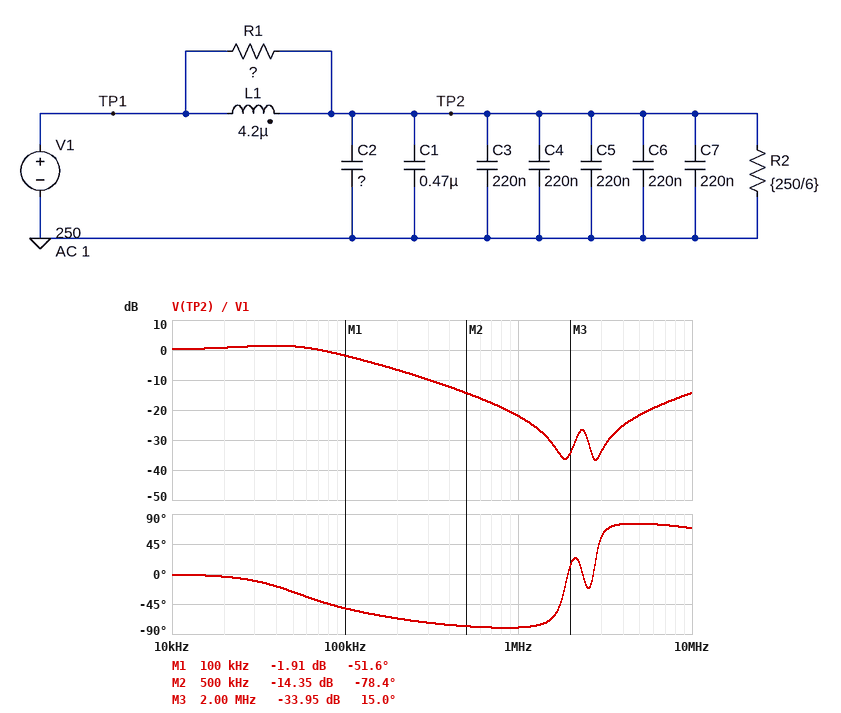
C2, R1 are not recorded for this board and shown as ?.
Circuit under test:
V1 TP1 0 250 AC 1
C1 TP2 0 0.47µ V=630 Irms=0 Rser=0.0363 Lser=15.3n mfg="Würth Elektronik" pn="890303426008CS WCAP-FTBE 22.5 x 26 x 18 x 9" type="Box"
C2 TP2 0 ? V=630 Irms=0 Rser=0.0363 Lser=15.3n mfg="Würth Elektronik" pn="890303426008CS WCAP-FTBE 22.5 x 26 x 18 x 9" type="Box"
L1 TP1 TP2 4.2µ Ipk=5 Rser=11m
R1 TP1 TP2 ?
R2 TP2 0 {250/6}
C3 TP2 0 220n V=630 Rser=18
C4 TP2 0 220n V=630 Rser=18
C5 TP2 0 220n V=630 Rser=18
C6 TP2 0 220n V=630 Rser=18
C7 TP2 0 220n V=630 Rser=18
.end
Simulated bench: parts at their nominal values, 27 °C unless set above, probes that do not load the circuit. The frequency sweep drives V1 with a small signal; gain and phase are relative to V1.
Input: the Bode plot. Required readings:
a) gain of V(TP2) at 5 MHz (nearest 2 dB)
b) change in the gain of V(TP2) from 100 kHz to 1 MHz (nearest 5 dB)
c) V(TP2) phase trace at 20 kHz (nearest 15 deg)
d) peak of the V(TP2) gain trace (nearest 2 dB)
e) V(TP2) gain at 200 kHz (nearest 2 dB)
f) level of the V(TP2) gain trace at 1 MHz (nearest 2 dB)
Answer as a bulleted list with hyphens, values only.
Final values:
- -22 dB
- -20 dB
- 0 deg
- 2 dB
- -6 dB
- -22 dB
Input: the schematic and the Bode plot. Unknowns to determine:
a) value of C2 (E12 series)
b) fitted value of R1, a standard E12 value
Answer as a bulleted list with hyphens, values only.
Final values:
- 220 nF
- 2.2 Ω
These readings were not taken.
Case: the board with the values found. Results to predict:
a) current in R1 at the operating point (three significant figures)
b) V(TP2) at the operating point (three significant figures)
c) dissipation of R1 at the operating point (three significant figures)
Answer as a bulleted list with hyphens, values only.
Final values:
- 29.8 mA
- 250 V
- 1.96 mW
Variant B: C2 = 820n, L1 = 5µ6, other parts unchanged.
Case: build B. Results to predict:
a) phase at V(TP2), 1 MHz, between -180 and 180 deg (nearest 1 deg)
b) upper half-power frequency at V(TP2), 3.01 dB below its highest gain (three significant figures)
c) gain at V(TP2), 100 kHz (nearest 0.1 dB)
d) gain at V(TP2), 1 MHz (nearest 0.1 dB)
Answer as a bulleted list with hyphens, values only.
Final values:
- -74 deg
- 62.3 kHz
- -5.1 dB
- -29.6 dB
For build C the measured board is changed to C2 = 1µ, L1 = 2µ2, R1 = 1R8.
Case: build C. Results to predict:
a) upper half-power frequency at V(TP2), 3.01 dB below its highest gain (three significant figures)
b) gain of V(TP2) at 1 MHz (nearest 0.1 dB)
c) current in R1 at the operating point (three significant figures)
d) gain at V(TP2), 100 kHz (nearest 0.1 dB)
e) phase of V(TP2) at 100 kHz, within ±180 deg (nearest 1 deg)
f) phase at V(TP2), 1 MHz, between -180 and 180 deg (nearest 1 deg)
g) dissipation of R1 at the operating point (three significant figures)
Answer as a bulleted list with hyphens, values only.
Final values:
- 102 kHz
- -30.1 dB
- 36.4 mA
- 0.2 dB
- -72 deg
- -70 deg
- 2.39 mW
